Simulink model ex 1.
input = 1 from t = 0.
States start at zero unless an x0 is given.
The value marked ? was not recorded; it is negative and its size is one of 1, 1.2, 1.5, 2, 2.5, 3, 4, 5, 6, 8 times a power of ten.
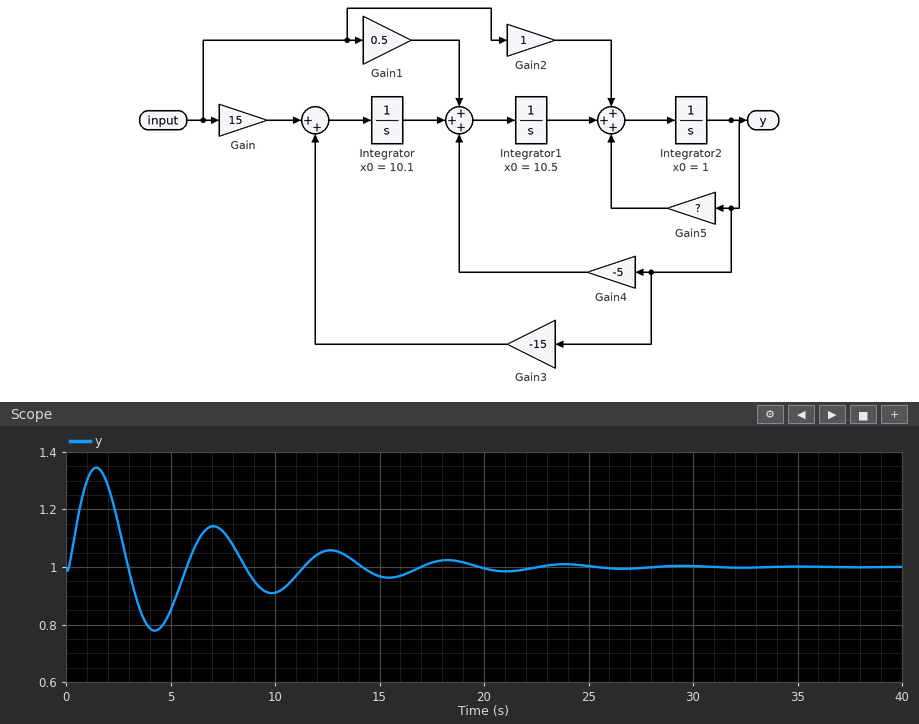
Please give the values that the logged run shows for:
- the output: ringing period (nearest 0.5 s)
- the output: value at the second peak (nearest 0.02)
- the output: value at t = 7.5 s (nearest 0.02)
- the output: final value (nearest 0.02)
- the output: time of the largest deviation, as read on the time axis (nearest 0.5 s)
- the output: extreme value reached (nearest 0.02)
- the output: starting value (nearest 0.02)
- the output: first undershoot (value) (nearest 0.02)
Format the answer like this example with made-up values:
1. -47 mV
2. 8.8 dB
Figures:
1. 5.5 s
2. 1.14
3. 1.12
4. 1.00
5. 1.5 s
6. 1.34
7. 1.00
8. 0.78
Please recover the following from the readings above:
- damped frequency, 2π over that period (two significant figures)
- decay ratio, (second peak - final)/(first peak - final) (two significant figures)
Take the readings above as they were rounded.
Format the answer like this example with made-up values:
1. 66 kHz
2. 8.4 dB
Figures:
1. 1.1 rad/s
2. 0.41
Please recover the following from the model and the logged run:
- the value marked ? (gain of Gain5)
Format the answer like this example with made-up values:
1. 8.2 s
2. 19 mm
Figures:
1. -12
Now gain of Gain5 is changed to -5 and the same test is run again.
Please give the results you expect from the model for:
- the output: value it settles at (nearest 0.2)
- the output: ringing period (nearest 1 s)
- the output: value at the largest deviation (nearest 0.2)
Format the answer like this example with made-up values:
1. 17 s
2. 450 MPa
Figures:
1. 1.0
2. 3 s
3. 2.2
